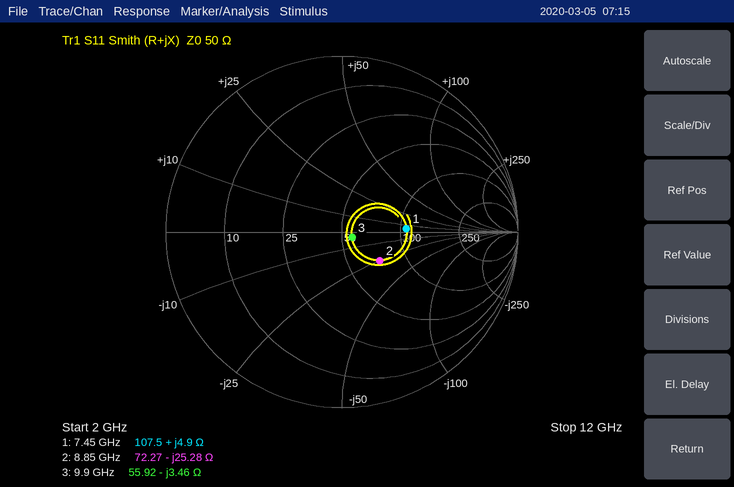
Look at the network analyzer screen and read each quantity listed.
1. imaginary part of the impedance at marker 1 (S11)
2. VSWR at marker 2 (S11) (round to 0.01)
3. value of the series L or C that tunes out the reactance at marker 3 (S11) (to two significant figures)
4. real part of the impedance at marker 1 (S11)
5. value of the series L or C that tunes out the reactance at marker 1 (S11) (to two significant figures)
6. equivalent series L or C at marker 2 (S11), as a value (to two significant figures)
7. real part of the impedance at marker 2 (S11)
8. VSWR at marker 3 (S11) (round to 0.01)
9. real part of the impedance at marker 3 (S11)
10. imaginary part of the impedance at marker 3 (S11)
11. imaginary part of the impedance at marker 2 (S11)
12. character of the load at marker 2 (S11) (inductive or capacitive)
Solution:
+4.9 Ω
1.74
56 pH
107.5 Ω
4.4 pF
710 fF
72.27 Ω
1.14
55.92 Ω
-3.46 Ω
-25.28 Ω
capacitive
